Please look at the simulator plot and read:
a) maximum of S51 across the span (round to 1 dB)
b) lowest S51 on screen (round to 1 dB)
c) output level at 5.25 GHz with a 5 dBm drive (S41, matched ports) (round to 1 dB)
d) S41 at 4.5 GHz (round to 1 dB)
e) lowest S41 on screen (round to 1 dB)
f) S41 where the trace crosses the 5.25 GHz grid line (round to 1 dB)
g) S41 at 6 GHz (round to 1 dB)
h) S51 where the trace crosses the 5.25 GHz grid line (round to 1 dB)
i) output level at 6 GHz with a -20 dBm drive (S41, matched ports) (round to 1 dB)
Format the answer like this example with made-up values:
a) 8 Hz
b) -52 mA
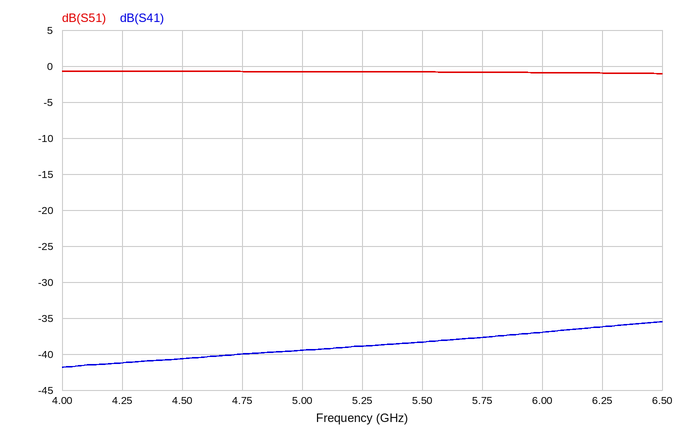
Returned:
a) -1 dB
b) -1 dB
c) -34 dBm
d) -41 dB
e) -42 dB
f) -39 dB
g) -37 dB
h) -1 dB
i) -57 dBm
